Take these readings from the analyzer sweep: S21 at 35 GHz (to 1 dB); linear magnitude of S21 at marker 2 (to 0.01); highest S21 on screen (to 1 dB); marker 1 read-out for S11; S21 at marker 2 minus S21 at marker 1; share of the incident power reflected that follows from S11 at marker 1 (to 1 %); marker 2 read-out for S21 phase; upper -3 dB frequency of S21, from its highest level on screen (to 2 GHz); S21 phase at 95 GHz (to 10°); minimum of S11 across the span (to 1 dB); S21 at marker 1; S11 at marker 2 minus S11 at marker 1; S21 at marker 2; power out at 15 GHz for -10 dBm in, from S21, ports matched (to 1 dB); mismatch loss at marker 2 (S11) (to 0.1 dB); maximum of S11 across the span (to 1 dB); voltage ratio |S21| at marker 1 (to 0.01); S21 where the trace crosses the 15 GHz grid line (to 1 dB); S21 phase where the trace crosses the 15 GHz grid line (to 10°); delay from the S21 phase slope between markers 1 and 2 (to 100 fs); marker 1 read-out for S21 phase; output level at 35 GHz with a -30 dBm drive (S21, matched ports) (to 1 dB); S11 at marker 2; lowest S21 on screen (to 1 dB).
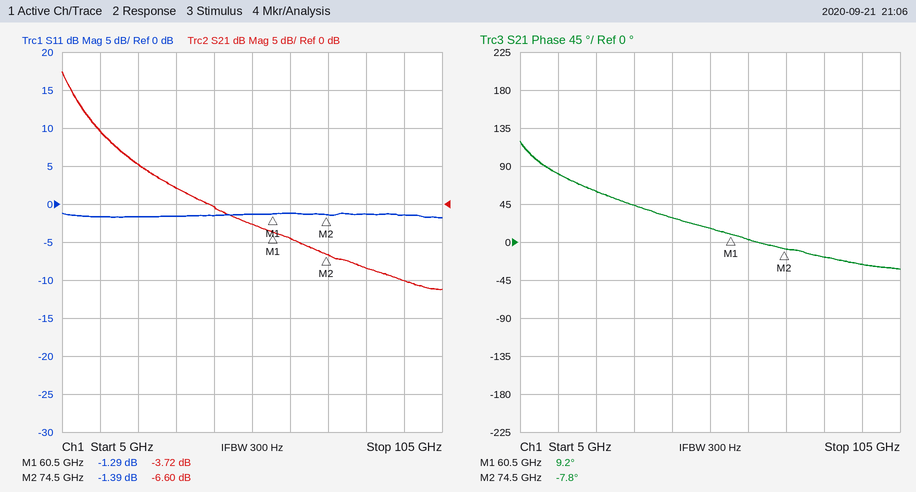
2 dB
0.47
17 dB
-1.29 dB
-2.88 dB
74 %
-7.8°
8 GHz
-30°
-2 dB
-3.72 dB
-0.10 dB
-6.60 dB
0 dBm
5.6 dB
-1 dB
0.65
10 dB
80°
3.4 ps
9.2°
-28 dBm
-1.39 dB
-11 dB
